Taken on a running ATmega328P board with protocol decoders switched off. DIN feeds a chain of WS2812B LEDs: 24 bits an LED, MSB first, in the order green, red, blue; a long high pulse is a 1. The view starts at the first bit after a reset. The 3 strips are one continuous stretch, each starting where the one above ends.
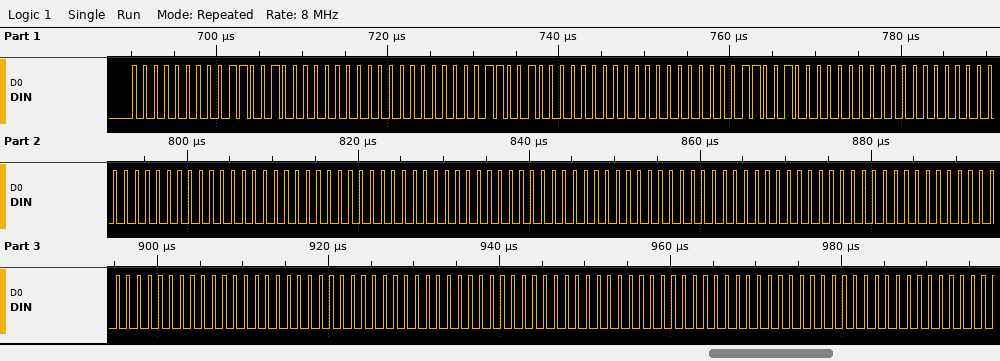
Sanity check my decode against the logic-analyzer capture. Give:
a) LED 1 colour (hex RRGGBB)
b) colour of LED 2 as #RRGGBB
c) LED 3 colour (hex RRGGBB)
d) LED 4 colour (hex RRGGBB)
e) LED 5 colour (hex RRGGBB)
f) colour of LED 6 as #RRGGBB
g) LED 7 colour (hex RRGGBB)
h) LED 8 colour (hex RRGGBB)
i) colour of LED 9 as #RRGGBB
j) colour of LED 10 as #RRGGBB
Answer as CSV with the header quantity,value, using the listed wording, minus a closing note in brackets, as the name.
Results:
quantity,value
LED 1 colour,#640000
colour of LED 2 as #RRGGBB,#640000
LED 3 colour,#640000
LED 4 colour,#000000
LED 5 colour,#000000
colour of LED 6 as #RRGGBB,#000000
LED 7 colour,#000000
LED 8 colour,#000000
colour of LED 9 as #RRGGBB,#000000
colour of LED 10 as #RRGGBB,#000000
